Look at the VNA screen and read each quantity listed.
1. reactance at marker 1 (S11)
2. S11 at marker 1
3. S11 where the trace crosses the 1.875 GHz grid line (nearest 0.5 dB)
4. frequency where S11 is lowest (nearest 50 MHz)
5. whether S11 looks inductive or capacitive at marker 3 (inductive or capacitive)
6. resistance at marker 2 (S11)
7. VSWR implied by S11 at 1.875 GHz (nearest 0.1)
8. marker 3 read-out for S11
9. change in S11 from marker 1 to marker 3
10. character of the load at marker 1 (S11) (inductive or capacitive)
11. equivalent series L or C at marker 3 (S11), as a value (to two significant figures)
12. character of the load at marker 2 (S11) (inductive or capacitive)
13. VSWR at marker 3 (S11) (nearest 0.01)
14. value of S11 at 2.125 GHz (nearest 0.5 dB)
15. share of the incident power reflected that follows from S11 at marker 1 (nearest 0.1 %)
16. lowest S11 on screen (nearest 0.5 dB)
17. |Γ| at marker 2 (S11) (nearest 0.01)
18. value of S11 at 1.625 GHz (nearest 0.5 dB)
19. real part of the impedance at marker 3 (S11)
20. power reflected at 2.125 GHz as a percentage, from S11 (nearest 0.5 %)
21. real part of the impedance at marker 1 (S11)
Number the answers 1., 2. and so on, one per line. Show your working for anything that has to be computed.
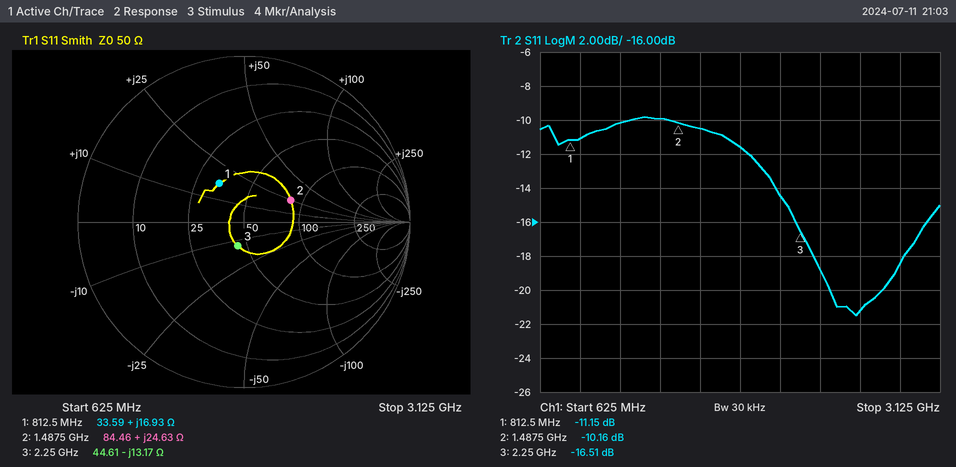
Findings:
1. +16.93 Ω
2. -11.15 dB
3. -11.5 dB
4. 2.60 GHz
5. capacitive
6. 84.46 Ω
7. |Γ| = 10^(-11.5/20) = 0.2661; VSWR = (1 + 0.2661)/(1 − 0.2661) ≈ 1.7
8. -16.51 dB
9. -16.51 − (-11.15) = -5.36 dB
10. inductive
11. C = 1/(2π × 2.25 GHz × 13.17 Ω) ≈ 5.4 pF
12. inductive
13. 1.35
14. -14.5 dB
15. 10^(-11.15/10) ≈ 7.7 %
16. -21.5 dB
17. 0.31
18. -10.5 dB
19. 44.61 Ω
20. 10^(-14.5/10) ≈ 3.5 %
21. 33.59 Ω
